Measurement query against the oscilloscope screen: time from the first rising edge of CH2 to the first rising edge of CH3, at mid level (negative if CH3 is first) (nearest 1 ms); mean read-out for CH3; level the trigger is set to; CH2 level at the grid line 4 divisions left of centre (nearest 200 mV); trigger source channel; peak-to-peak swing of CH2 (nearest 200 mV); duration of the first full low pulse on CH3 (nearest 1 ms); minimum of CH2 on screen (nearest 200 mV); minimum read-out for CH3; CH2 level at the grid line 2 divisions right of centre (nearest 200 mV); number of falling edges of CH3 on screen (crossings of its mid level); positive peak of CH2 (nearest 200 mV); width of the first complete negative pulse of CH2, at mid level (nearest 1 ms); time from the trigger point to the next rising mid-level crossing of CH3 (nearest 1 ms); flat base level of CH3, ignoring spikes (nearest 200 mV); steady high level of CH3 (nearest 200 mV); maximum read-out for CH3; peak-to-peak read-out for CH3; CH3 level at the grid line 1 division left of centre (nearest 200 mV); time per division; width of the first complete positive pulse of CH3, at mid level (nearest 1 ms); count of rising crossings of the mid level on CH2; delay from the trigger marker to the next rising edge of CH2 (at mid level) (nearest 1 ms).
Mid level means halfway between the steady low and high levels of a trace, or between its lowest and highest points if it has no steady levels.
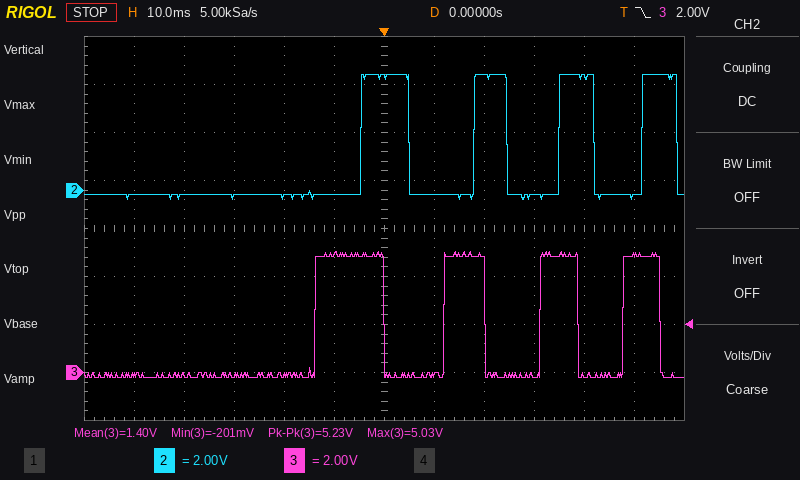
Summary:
-9 ms
1.40 V
2.00 V
-200 mV
CH3
5.2 V
12 ms
-400 mV
-201 mV
4.8 V
4
4.8 V
13 ms
12 ms
-200 mV
4.8 V
5.03 V
5.23 V
5.0 V
10 ms
14 ms
4
18 ms
